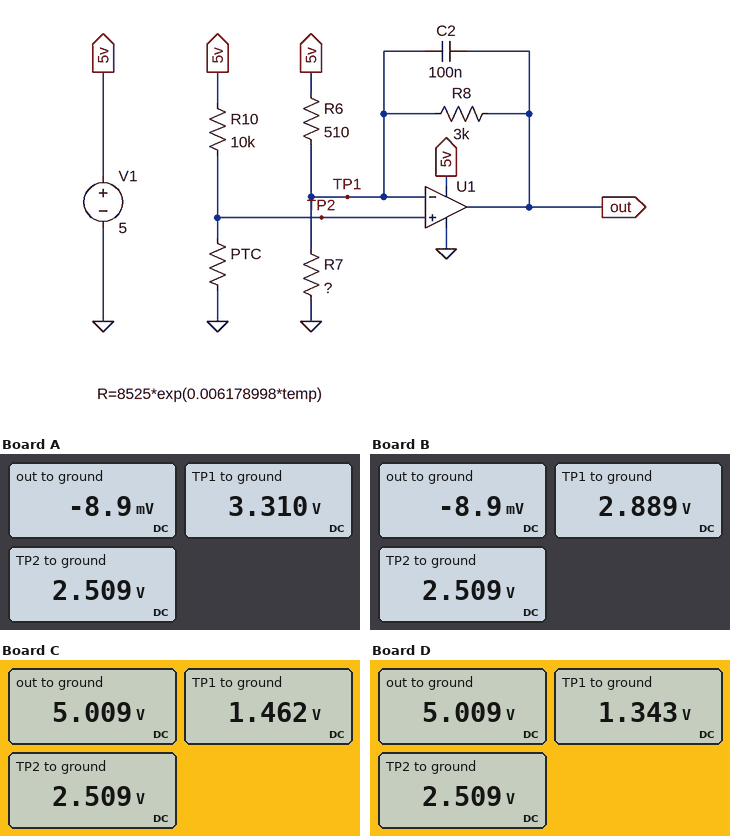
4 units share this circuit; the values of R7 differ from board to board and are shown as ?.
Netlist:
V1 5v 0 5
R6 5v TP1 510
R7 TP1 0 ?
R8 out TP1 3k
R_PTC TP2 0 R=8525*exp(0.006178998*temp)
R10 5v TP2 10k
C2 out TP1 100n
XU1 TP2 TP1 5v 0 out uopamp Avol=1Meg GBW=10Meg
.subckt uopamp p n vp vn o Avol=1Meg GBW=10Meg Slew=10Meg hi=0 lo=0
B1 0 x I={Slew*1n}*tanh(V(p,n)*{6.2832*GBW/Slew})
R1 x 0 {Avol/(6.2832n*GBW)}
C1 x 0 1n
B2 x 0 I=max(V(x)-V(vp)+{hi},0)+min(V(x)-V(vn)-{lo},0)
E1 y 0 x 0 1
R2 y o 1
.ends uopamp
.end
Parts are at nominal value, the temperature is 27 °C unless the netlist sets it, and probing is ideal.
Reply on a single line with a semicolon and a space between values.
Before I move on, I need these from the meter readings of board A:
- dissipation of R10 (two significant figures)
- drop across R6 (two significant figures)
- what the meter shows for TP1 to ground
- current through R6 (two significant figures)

620 µW; 1.7 V; 3.310 V; 3.3 mA
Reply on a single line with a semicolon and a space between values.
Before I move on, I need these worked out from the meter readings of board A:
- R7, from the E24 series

1.5 kΩ
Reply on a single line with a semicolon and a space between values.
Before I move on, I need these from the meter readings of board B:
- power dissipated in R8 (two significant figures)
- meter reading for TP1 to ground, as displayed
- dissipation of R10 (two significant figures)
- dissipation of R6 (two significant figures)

2.8 mW; 2.889 V; 620 µW; 8.7 mW
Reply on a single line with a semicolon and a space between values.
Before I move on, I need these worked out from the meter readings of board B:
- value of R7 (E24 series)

910 Ω
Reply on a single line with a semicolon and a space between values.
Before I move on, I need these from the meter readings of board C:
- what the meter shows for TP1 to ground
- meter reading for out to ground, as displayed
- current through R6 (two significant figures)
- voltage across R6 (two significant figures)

1.462 V; 5.009 V; 6.9 mA; 3.5 V
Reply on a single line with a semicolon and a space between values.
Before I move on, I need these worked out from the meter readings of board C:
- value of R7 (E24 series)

180 Ω
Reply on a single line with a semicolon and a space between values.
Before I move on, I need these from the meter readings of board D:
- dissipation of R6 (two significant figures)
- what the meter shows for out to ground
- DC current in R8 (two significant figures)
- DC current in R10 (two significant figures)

26 mW; 5.009 V; 1.2 mA; 250 µA
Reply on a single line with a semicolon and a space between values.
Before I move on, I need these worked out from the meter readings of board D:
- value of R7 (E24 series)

160 Ω
